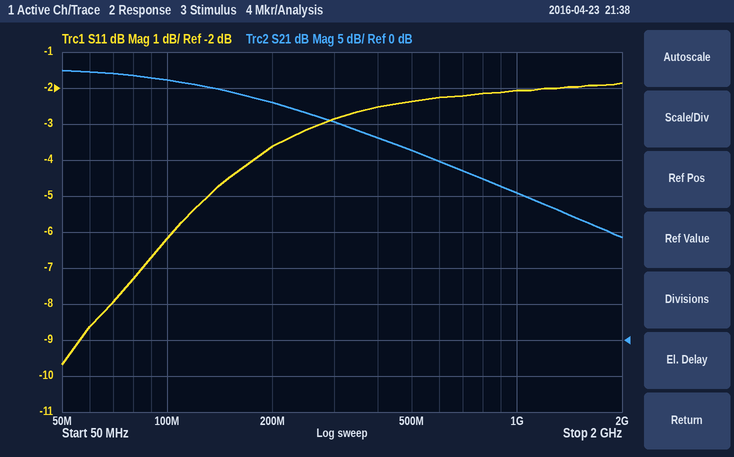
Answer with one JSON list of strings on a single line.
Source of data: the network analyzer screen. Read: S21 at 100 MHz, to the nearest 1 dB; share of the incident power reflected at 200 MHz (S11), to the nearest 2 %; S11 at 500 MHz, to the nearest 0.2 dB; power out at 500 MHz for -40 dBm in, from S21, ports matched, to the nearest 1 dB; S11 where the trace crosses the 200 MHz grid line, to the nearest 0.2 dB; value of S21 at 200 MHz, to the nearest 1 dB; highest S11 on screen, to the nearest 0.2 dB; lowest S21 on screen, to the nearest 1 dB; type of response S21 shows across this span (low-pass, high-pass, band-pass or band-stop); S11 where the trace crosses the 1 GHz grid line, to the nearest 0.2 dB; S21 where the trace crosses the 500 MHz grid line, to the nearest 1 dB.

["36 dB", "44 %", "-2.4 dB", "-14 dBm", "-3.6 dB", "33 dB", "-1.8 dB", "14 dB", "low-pass", "-2.0 dB", "26 dB"]
